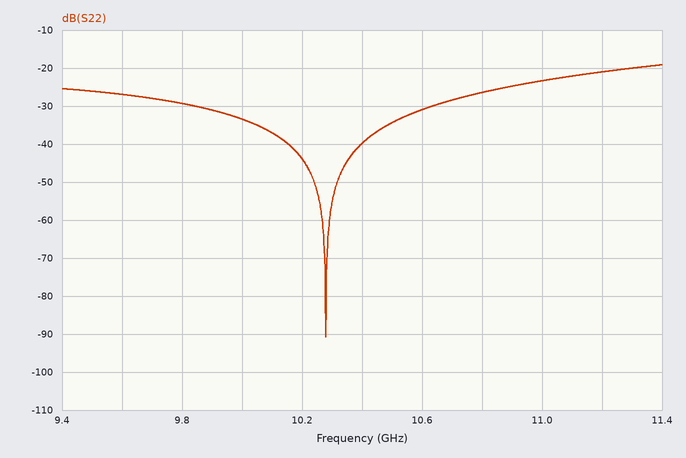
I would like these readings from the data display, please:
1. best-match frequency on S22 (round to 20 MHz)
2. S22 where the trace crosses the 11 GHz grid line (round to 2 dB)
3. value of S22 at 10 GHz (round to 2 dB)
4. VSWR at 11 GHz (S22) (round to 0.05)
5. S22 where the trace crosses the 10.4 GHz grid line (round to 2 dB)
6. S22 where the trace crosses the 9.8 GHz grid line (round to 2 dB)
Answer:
10.28 GHz
-24 dB
-34 dB
1.15
-40 dB
-30 dB
